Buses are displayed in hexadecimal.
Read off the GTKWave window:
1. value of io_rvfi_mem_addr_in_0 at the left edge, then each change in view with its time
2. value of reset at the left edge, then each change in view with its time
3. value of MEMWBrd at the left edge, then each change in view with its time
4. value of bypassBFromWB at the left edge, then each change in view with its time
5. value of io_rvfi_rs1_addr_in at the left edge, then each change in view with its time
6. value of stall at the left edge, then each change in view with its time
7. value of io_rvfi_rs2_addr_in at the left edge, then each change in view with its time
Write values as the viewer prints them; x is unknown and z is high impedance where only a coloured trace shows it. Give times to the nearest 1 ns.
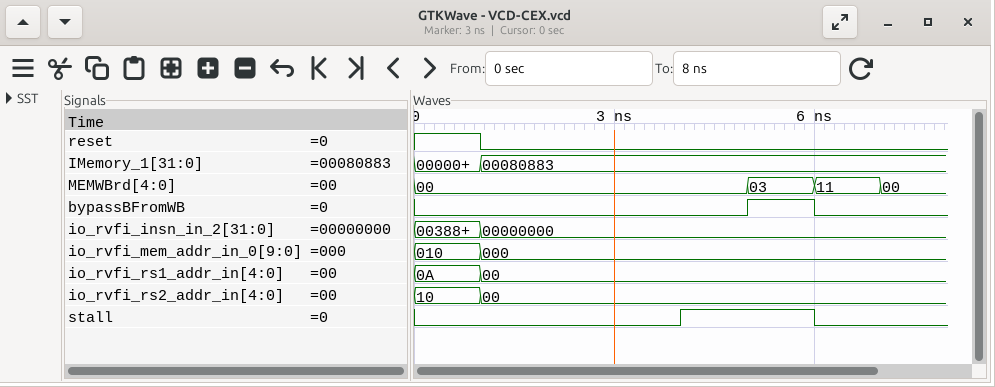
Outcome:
010, 000 at 1 ns
1, 0 at 1 ns
00, 03 at 5 ns, 11 at 6 ns, 00 at 7 ns
0, 1 at 5 ns, 0 at 6 ns
0A, 00 at 1 ns
0, 1 at 4 ns, 0 at 6 ns
10, 00 at 1 ns
